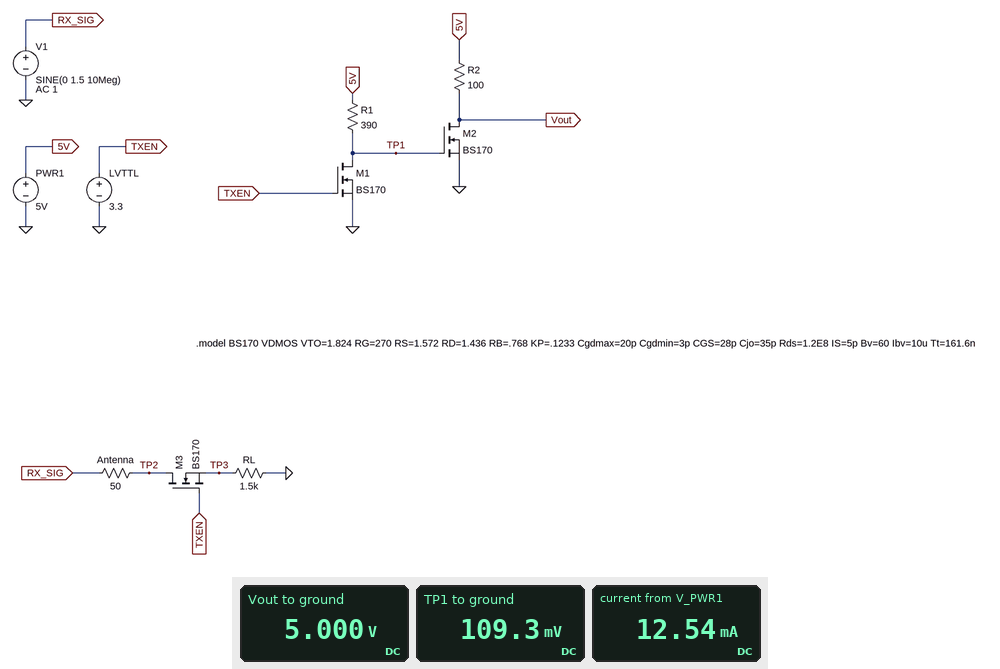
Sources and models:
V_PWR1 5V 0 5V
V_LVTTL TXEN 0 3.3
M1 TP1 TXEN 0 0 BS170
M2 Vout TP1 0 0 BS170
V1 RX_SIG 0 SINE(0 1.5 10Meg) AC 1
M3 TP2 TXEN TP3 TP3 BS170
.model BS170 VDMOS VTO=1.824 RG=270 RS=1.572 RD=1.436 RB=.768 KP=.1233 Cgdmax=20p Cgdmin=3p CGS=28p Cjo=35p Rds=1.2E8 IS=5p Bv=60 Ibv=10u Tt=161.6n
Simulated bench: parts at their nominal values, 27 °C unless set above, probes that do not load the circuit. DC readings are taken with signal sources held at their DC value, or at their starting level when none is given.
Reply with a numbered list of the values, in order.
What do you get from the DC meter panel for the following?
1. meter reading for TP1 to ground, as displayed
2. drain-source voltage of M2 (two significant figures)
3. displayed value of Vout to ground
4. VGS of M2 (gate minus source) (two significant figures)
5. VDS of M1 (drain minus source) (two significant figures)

1. 109.3 mV
2. 5.0 V
3. 5.000 V
4. 110 mV
5. 110 mV
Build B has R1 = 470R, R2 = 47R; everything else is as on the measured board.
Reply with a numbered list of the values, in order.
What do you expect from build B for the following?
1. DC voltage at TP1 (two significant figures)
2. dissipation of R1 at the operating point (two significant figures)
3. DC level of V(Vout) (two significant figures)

1. 91 mV
2. 51 mW
3. 5.0 V
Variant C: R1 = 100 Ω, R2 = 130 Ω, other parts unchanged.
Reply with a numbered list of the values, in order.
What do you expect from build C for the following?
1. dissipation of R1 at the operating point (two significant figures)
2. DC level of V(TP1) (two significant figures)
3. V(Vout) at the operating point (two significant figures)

1. 210 mW
2. 430 mV
3. 5.0 V
